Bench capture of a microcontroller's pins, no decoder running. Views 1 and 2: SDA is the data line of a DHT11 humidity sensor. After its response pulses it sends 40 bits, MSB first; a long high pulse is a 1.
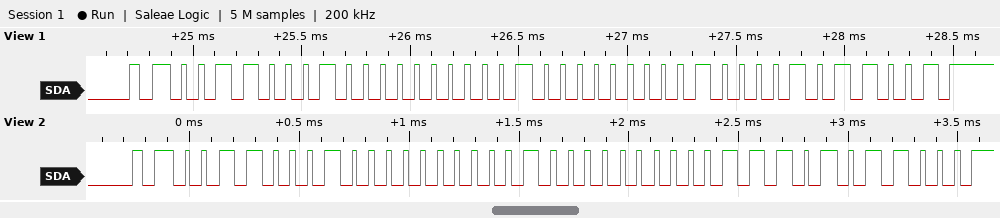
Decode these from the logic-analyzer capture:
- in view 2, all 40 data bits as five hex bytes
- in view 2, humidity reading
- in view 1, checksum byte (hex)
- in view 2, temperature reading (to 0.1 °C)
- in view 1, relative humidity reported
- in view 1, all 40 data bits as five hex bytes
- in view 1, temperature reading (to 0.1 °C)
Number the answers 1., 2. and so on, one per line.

1. 31 00 20 07 58
2. 49 %
3. 0x59
4. 32.7 °C
5. 49 %
6. 31 00 20 08 59
7. 32.8 °C
